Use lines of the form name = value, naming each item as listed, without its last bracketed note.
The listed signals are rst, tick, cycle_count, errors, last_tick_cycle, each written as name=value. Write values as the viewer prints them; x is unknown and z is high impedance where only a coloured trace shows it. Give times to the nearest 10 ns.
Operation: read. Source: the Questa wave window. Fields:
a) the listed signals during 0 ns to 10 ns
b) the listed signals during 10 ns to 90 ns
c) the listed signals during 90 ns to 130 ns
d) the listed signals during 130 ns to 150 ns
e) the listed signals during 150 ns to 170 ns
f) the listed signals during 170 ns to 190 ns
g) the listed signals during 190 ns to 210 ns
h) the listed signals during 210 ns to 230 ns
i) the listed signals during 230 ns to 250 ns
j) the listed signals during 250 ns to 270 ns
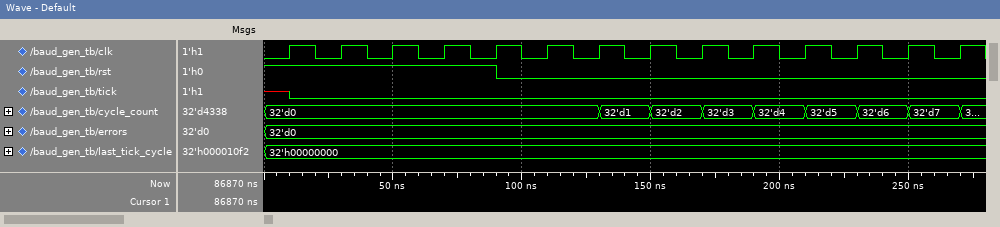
the listed signals during 0 ns to 10 ns = rst=1, tick=x, cycle_count=32'd0, errors=32'd0, last_tick_cycle=32'h00000000
the listed signals during 10 ns to 90 ns = rst=1, tick=0, cycle_count=32'd0, errors=32'd0, last_tick_cycle=32'h00000000
the listed signals during 90 ns to 130 ns = rst=0, tick=0, cycle_count=32'd0, errors=32'd0, last_tick_cycle=32'h00000000
the listed signals during 130 ns to 150 ns = rst=0, tick=0, cycle_count=32'd1, errors=32'd0, last_tick_cycle=32'h00000000
the listed signals during 150 ns to 170 ns = rst=0, tick=0, cycle_count=32'd2, errors=32'd0, last_tick_cycle=32'h00000000
the listed signals during 170 ns to 190 ns = rst=0, tick=0, cycle_count=32'd3, errors=32'd0, last_tick_cycle=32'h00000000
the listed signals during 190 ns to 210 ns = rst=0, tick=0, cycle_count=32'd4, errors=32'd0, last_tick_cycle=32'h00000000
the listed signals during 210 ns to 230 ns = rst=0, tick=0, cycle_count=32'd5, errors=32'd0, last_tick_cycle=32'h00000000
the listed signals during 230 ns to 250 ns = rst=0, tick=0, cycle_count=32'd6, errors=32'd0, last_tick_cycle=32'h00000000
the listed signals during 250 ns to 270 ns = rst=0, tick=0, cycle_count=32'd7, errors=32'd0, last_tick_cycle=32'h00000000
